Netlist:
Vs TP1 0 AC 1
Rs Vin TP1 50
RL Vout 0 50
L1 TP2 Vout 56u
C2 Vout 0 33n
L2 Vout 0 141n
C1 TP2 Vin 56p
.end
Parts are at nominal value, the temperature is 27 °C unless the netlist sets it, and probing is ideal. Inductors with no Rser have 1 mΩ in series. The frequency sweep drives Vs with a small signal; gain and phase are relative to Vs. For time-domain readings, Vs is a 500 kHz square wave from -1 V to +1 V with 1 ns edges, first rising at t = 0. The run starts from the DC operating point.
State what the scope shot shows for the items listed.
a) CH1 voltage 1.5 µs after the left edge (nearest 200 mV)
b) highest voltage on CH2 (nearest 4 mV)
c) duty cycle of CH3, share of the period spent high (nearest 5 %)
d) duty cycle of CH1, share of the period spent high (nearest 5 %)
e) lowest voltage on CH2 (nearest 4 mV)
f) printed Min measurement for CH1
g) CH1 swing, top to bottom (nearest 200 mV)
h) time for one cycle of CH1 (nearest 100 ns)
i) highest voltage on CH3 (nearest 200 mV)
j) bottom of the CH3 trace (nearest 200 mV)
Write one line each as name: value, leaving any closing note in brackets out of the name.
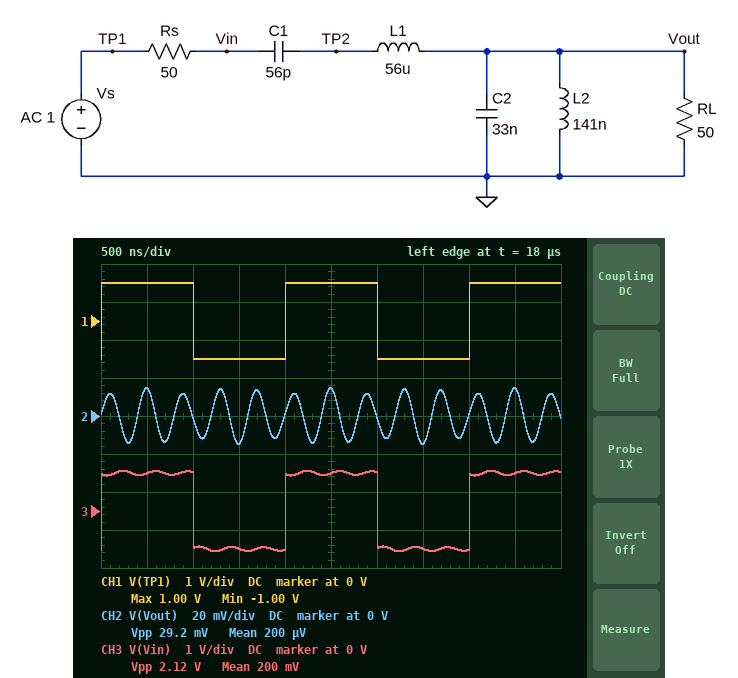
CH1 voltage 1.5 µs after the left edge: -1.0 V
highest voltage on CH2: 16 mV
duty cycle of CH3, share of the period spent high: 50 %
duty cycle of CH1, share of the period spent high: 50 %
lowest voltage on CH2: -16 mV
printed Min measurement for CH1: -1.00 V
CH1 swing, top to bottom: 2.0 V
time for one cycle of CH1: 2.0 µs
highest voltage on CH3: 1.0 V
bottom of the CH3 trace: -1.0 V
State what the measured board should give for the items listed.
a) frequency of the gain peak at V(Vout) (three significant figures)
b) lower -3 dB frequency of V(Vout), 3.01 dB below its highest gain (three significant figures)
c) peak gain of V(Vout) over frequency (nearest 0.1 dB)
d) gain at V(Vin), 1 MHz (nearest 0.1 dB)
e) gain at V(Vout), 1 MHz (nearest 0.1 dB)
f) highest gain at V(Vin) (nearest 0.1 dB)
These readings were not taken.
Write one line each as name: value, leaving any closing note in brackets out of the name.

frequency of the gain peak at V(Vout): 2.33 MHz
lower -3 dB frequency of V(Vout), 3.01 dB below its highest gain: 2.29 MHz
peak gain of V(Vout) over frequency: -18.4 dB
gain at V(Vin), 1 MHz: 0 dB
gain at V(Vout), 1 MHz: -67.2 dB
highest gain at V(Vin): 0 dB
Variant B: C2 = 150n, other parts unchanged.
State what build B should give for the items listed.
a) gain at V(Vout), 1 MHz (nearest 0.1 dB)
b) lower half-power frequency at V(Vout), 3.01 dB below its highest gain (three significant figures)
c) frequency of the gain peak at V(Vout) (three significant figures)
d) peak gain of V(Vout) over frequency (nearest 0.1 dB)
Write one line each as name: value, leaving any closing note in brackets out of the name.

gain at V(Vout), 1 MHz: -53.4 dB
lower half-power frequency at V(Vout), 3.01 dB below its highest gain: 1.08 MHz
frequency of the gain peak at V(Vout): 1.09 MHz
peak gain of V(Vout) over frequency: -33.4 dB
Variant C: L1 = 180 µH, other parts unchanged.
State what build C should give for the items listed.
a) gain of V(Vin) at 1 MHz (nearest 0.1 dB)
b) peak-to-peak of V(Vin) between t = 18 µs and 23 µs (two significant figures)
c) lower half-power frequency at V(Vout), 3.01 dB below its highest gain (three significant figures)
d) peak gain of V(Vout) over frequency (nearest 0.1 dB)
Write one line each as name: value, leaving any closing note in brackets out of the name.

gain of V(Vin) at 1 MHz: 0 dB
peak-to-peak of V(Vin) between t = 18 µs and 23 µs: 2.2 V
lower half-power frequency at V(Vout), 3.01 dB below its highest gain: 1.56 MHz
peak gain of V(Vout) over frequency: -25.7 dB
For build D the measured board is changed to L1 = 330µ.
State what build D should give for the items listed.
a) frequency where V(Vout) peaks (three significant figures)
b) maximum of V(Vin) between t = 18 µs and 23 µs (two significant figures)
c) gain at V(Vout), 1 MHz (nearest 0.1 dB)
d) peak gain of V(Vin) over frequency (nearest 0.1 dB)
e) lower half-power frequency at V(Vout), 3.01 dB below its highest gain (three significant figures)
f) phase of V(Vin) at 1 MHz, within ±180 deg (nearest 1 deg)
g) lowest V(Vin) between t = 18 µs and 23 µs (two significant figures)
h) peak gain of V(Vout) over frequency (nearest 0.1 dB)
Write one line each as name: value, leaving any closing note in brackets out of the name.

frequency where V(Vout) peaks: 1.17 MHz
maximum of V(Vin) between t = 18 µs and 23 µs: 1.0 V
gain at V(Vout), 1 MHz: -57.0 dB
peak gain of V(Vin) over frequency: 0 dB
lower half-power frequency at V(Vout), 3.01 dB below its highest gain: 1.16 MHz
phase of V(Vin) at 1 MHz, within ±180 deg: -4 deg
lowest V(Vin) between t = 18 µs and 23 µs: -1.0 V
peak gain of V(Vout) over frequency: -31.2 dB
